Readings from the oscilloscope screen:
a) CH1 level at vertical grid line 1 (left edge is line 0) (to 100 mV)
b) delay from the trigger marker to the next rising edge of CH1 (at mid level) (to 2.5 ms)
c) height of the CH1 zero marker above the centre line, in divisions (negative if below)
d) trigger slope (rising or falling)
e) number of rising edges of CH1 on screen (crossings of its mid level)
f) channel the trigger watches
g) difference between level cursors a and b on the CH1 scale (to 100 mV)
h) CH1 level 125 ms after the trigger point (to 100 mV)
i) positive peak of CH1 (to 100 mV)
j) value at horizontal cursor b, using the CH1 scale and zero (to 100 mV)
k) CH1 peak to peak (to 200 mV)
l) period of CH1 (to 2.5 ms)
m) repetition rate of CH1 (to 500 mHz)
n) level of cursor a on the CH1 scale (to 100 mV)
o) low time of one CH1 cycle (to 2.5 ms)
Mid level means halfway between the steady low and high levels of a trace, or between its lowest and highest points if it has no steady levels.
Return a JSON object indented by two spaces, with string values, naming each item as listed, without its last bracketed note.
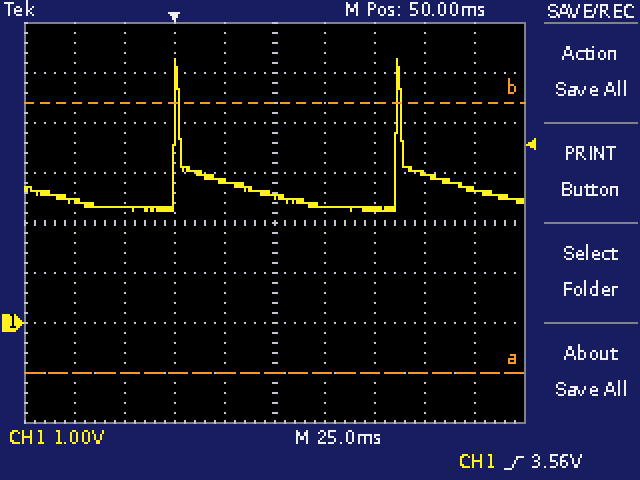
{
  "CH1 level at vertical grid line 1 (left edge is line 0)": "2.4 V",
  "delay from the trigger marker to the next rising edge of CH1 (at mid level)": "110.0 ms",
  "height of the CH1 zero marker above the centre line, in divisions": "-2.0 div",
  "trigger slope": "rising",
  "number of rising edges of CH1 on screen": "2",
  "channel the trigger watches": "CH1",
  "difference between level cursors a and b on the CH1 scale": "5.4 V",
  "CH1 level 125 ms after the trigger point": "3.0 V",
  "positive peak of CH1": "5.3 V",
  "value at horizontal cursor b, using the CH1 scale and zero": "4.4 V",
  "CH1 peak to peak": "3.0 V",
  "period of CH1": "110.0 ms",
  "repetition rate of CH1": "9.0 Hz",
  "level of cursor a on the CH1 scale": "-1.0 V",
  "low time of one CH1 cycle": "107.5 ms"
}
